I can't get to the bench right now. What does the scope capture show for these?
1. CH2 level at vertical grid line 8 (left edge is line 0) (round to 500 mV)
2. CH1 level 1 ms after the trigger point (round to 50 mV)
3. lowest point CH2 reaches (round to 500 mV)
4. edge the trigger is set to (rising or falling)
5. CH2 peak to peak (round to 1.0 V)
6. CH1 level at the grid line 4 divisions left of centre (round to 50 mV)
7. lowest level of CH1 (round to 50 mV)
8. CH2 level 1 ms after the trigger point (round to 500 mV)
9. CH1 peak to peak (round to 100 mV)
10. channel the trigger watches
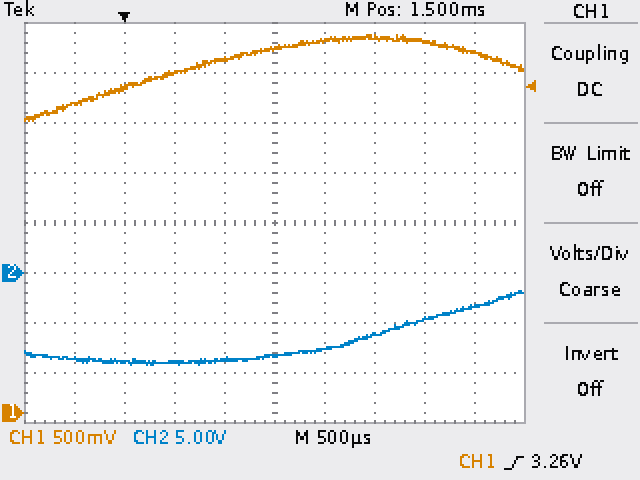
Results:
-4.5 V
3.55 V
-9.0 V
rising
7.0 V
3.10 V
2.90 V
-8.5 V
900 mV
CH1
